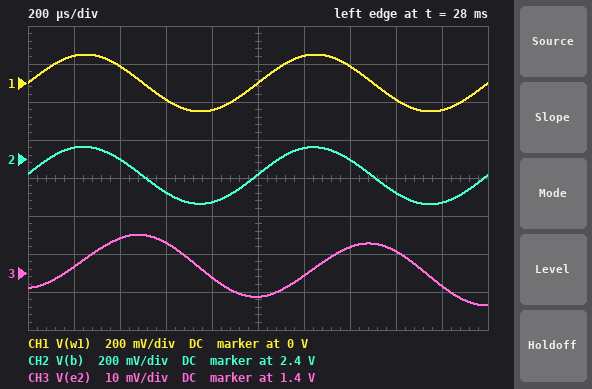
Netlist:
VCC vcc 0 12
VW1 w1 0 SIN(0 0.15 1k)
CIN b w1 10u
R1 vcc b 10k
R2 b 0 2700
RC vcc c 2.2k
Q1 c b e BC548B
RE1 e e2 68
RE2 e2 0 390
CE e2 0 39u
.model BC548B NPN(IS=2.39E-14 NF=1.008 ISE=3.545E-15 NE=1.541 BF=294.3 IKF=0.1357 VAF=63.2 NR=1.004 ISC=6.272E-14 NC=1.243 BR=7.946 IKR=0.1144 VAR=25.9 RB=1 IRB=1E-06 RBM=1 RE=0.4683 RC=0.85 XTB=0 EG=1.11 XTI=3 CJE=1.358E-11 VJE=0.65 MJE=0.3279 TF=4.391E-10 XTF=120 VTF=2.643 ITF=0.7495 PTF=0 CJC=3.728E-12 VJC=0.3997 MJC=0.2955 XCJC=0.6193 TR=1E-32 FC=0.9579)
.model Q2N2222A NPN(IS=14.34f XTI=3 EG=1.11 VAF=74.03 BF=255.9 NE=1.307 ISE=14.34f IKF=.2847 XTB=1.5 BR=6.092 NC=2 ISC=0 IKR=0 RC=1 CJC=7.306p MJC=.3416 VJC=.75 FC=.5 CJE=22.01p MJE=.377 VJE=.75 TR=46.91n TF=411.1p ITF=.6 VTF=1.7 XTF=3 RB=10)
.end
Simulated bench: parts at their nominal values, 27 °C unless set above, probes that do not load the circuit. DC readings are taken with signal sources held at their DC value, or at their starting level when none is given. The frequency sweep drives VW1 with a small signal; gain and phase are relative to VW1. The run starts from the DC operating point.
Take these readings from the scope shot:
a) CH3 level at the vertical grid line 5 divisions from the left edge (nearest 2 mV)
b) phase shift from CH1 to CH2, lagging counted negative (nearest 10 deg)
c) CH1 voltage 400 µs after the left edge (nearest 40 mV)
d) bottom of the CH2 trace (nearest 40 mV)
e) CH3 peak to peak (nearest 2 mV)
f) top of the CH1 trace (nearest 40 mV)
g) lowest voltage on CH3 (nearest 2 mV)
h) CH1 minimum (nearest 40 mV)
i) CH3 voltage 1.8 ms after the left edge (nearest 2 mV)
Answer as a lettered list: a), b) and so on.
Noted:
a) 1.394 V
b) 0 deg
c) 80 mV
d) 2.16 V
e) 18 mV
f) 160 mV
g) 1.392 V
h) -160 mV
i) 1.396 V
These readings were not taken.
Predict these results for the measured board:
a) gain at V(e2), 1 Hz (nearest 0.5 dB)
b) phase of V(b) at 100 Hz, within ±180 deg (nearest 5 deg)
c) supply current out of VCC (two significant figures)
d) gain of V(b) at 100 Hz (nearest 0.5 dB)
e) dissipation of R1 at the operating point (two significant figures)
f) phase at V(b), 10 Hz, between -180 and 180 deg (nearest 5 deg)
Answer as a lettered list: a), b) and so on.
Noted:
a) -19.5 dB
b) 5 deg
c) 5.0 mA
d) 0 dB
e) 9.0 mW
f) 35 deg
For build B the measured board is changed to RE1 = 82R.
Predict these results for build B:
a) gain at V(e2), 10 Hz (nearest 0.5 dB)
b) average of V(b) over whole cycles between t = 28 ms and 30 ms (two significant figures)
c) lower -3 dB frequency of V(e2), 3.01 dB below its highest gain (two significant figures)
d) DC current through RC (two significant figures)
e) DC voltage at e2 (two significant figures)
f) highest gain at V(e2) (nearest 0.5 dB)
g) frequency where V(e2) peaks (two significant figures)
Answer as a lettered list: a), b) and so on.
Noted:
a) -4.0 dB
b) 2.4 V
c) 6.1 Hz
d) 3.9 mA
e) 1.5 V
f) -3.0 dB
g) 21 Hz
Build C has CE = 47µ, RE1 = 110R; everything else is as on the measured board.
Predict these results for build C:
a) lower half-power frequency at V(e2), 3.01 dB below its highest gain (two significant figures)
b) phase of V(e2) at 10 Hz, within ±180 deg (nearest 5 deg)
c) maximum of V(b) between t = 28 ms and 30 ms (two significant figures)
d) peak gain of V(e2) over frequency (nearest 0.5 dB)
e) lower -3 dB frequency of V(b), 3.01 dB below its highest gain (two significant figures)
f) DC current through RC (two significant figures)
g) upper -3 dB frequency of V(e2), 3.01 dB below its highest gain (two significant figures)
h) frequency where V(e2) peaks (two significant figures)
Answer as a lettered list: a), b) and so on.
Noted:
a) 5.6 Hz
b) 20 deg
c) 2.6 V
d) -4.0 dB
e) 7.7 Hz
f) 3.7 mA
g) 51 Hz
h) 17 Hz
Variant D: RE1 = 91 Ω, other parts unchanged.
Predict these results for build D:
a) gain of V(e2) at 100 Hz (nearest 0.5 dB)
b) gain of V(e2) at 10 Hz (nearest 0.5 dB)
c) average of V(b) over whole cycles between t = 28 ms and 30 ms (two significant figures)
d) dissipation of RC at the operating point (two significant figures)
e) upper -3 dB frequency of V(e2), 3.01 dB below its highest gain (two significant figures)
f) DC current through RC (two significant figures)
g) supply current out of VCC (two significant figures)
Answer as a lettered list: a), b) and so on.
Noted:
a) -9.0 dB
b) -4.0 dB
c) 2.4 V
d) 32 mW
e) 66 Hz
f) 3.8 mA
g) 4.8 mA
